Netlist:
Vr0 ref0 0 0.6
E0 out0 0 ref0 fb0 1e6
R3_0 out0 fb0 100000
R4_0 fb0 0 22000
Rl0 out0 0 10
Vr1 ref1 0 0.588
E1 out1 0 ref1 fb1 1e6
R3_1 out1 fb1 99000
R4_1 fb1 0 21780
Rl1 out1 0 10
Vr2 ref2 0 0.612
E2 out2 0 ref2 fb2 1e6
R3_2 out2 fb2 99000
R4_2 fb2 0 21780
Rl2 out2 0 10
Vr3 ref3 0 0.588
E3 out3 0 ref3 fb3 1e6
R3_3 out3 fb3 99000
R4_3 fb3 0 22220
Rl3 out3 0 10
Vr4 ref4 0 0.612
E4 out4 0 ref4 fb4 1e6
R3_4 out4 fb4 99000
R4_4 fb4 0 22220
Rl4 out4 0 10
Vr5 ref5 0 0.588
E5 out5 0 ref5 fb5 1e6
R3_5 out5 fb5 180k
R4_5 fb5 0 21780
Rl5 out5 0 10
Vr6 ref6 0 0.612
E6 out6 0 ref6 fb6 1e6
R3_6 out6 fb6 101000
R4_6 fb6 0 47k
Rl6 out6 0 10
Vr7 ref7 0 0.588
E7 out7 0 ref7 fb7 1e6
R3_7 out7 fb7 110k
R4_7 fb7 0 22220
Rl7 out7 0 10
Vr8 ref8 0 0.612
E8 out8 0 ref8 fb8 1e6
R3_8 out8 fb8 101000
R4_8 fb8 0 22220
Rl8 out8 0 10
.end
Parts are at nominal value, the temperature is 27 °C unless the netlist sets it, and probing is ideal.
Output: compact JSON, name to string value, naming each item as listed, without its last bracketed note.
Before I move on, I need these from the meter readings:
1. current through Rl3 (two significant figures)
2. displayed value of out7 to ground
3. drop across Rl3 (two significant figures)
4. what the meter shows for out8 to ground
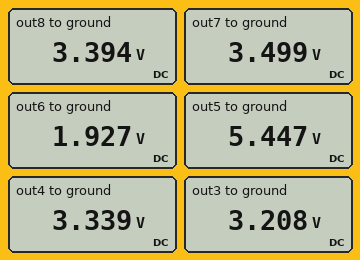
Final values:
{"current through Rl3": "320 mA", "displayed value of out7 to ground": "3.499 V", "drop across Rl3": "3.2 V", "what the meter shows for out8 to ground": "3.394 V"}
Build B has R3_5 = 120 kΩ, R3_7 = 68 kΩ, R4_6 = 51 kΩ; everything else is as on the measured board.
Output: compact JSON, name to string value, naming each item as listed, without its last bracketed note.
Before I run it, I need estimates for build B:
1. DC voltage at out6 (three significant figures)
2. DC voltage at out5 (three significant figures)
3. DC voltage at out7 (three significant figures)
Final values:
{"DC voltage at out6": "1.82 V", "DC voltage at out5": "3.83 V", "DC voltage at out7": "2.39 V"}
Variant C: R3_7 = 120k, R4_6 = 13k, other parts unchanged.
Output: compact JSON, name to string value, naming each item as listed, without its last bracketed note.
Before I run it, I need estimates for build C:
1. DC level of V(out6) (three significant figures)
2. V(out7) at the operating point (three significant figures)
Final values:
{"DC level of V(out6)": "5.37 V", "V(out7) at the operating point": "3.76 V"}
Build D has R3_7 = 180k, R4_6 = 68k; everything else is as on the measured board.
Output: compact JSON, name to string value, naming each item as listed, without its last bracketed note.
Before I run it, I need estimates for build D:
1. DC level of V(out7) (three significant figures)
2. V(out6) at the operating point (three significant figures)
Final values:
{"DC level of V(out7)": "5.35 V", "V(out6) at the operating point": "1.52 V"}
